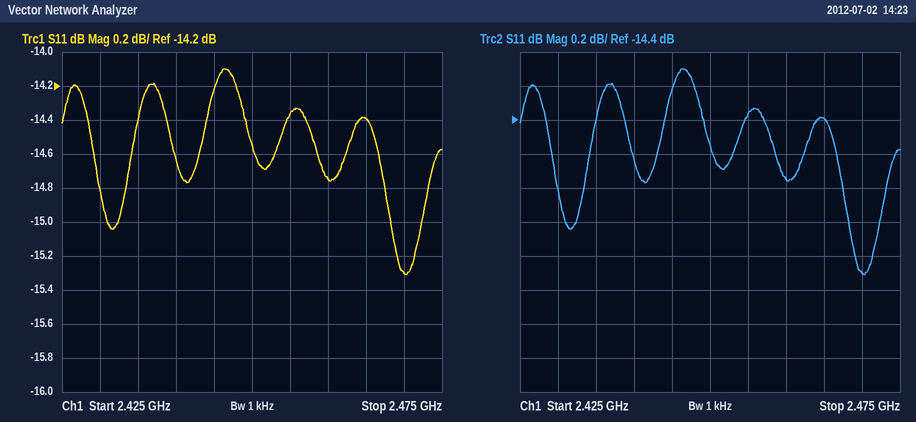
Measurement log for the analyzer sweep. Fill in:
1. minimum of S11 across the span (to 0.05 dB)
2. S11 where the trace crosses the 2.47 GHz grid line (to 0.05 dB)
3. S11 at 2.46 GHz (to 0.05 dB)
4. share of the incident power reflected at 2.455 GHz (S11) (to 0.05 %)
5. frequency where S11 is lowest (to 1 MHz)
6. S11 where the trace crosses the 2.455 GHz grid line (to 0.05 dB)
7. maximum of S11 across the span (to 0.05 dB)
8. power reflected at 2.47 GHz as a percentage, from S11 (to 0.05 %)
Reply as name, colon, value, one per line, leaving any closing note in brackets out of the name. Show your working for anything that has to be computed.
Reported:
minimum of S11 across the span: -15.30 dB
S11 where the trace crosses the 2.47 GHz grid line: -15.30 dB
S11 at 2.46 GHz: -14.75 dB
share of the incident power reflected at 2.455 GHz (S11): 10^(-14.35/10) ≈ 3.67 %, so 3.65 % to the nearest 0.05 %
frequency where S11 is lowest: 2.470 GHz
S11 where the trace crosses the 2.455 GHz grid line: -14.35 dB
maximum of S11 across the span: -14.10 dB
power reflected at 2.47 GHz as a percentage, from S11: 10^(-15.3/10) ≈ 2.95 %
